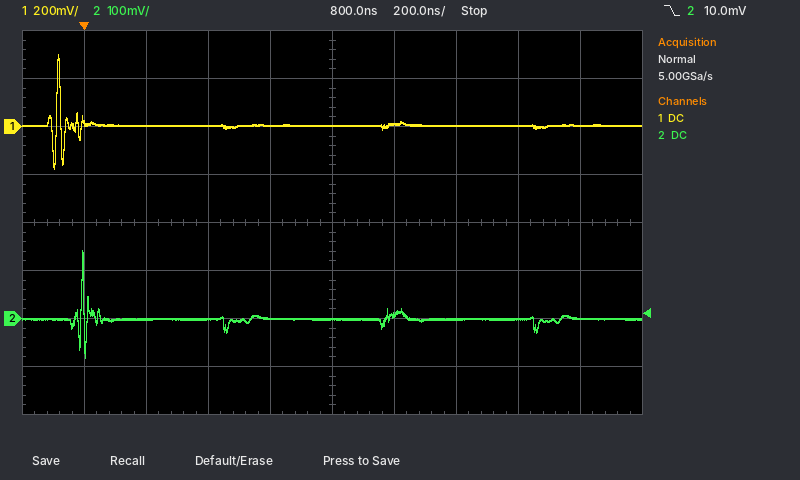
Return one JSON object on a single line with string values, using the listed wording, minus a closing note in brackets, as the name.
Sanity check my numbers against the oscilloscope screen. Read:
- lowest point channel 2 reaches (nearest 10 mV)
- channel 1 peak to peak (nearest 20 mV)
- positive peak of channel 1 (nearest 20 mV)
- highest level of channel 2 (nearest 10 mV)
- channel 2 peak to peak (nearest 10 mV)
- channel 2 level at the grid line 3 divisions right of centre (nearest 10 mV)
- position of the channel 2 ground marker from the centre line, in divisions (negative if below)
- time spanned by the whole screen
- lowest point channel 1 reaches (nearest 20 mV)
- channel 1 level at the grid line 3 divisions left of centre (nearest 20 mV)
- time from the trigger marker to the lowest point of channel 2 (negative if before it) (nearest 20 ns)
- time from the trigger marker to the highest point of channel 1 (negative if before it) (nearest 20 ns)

{"lowest point channel 2 reaches": "-80 mV", "channel 1 peak to peak": "480 mV", "positive peak of channel 1": "300 mV", "highest level of channel 2": "140 mV", "channel 2 peak to peak": "220 mV", "channel 2 level at the grid line 3 divisions right of centre": "0 mV", "position of the channel 2 ground marker from the centre line, in divisions": "-2.0 div", "time spanned by the whole screen": "2 µs", "lowest point channel 1 reaches": "-180 mV", "channel 1 level at the grid line 3 divisions left of centre": "0 mV", "time from the trigger marker to the lowest point of channel 2 (negative if before it)": "0 ns", "time from the trigger marker to the highest point of channel 1 (negative if before it)": "-80 ns"}
